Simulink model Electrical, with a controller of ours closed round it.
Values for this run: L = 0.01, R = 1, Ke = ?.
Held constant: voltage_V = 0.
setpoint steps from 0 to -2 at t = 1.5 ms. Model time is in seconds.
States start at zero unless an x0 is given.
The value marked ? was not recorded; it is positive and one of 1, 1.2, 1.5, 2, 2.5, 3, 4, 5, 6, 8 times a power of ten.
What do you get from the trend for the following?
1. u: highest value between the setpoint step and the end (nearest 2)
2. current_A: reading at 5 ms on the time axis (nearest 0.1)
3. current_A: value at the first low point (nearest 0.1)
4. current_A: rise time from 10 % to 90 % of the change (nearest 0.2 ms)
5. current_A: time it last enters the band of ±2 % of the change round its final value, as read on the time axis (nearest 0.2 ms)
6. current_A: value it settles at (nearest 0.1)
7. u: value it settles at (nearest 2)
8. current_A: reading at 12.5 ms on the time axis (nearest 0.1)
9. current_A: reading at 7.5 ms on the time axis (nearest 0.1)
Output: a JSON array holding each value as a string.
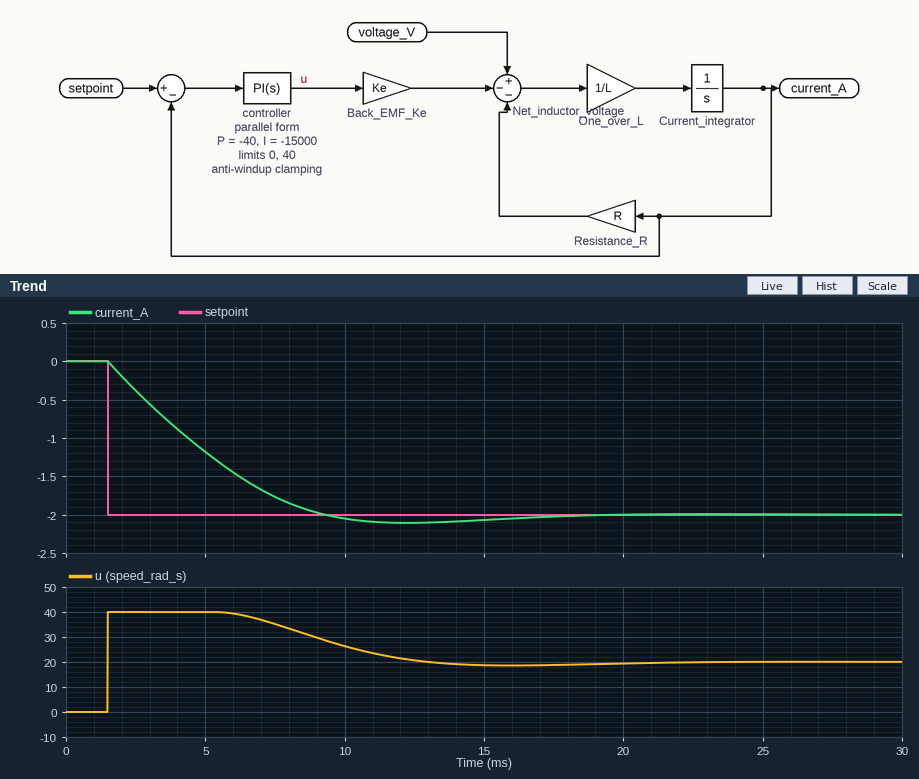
["40", "-1.2", "-2.1", "5.6 ms", "16.6 ms", "-2.0", "20", "-2.1", "-1.8"]
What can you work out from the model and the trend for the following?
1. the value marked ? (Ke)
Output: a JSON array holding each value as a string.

["0.1"]
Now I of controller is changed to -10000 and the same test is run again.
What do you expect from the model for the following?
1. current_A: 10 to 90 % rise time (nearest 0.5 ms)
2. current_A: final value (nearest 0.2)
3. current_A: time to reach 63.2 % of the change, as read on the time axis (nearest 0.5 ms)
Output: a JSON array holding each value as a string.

["6.5 ms", "-2.0", "5.5 ms"]
